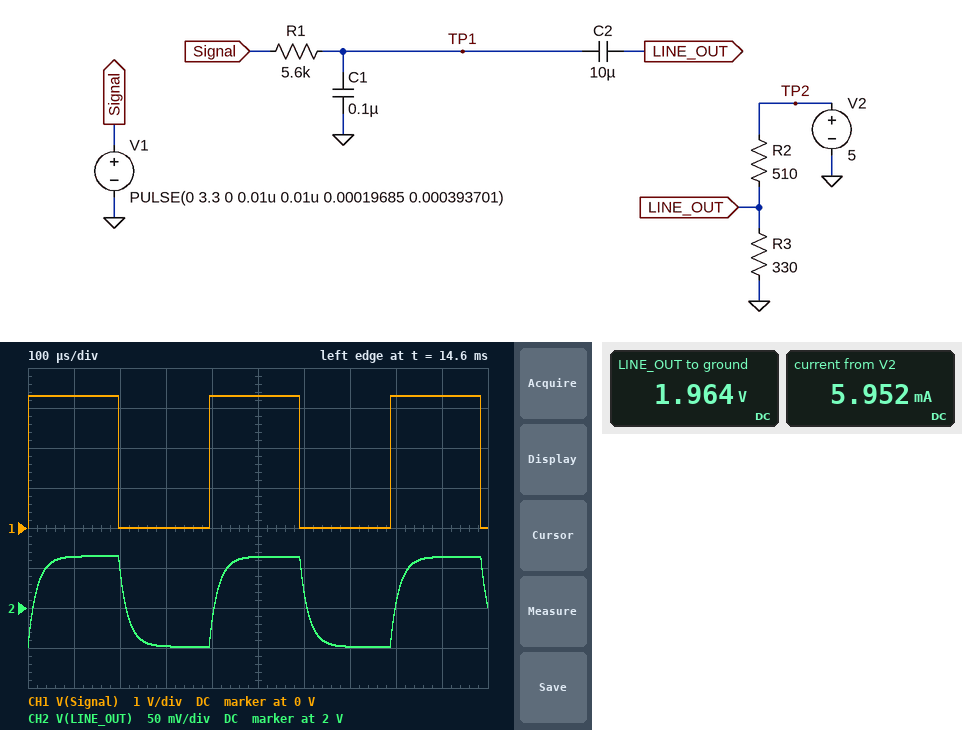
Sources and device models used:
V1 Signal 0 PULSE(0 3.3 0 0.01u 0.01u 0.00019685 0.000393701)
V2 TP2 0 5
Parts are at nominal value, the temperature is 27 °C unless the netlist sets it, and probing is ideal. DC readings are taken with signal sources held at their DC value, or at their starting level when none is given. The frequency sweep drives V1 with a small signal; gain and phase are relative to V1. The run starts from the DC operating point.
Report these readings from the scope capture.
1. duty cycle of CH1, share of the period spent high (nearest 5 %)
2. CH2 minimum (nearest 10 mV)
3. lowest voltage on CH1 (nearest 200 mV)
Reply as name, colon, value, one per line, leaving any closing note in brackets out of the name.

duty cycle of CH1, share of the period spent high: 50 %
CH2 minimum: 1.95 V
lowest voltage on CH1: 0 V
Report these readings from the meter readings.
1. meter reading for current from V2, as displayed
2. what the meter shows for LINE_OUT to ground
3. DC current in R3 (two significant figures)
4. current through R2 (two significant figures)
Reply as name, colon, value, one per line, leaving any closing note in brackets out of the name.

meter reading for current from V2, as displayed: 5.952 mA
what the meter shows for LINE_OUT to ground: 1.964 V
DC current in R3: 6.0 mA
current through R2: 6.0 mA
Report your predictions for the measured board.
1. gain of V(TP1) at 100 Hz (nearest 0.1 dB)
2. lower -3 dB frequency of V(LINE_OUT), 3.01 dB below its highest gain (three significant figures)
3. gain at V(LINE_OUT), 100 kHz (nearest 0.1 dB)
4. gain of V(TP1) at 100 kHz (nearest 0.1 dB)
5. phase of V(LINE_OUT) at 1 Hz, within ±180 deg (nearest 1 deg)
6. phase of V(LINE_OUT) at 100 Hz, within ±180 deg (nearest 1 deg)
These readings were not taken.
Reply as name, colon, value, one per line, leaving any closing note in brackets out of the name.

gain of V(TP1) at 100 Hz: -27.2 dB
lower -3 dB frequency of V(LINE_OUT), 3.01 dB below its highest gain: 2.72 Hz
gain at V(LINE_OUT), 100 kHz: -51.0 dB
gain of V(TP1) at 100 kHz: -51.0 dB
phase of V(LINE_OUT) at 1 Hz, within ±180 deg: 70 deg
phase of V(LINE_OUT) at 100 Hz, within ±180 deg: 1 deg
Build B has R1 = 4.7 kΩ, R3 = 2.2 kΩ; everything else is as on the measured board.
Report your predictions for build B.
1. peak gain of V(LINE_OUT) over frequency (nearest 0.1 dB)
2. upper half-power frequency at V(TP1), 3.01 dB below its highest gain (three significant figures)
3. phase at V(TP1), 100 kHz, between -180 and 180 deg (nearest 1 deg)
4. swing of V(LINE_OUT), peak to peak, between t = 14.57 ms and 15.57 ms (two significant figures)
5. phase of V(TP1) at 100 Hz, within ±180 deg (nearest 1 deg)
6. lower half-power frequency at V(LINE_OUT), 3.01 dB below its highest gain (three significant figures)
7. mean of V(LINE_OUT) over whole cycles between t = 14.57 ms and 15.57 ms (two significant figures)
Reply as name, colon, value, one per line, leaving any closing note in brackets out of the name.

peak gain of V(LINE_OUT) over frequency: -21.9 dB
upper half-power frequency at V(TP1), 3.01 dB below its highest gain: 3.11 Hz
phase at V(TP1), 100 kHz, between -180 and 180 deg: -88 deg
swing of V(LINE_OUT), peak to peak, between t = 14.57 ms and 15.57 ms: 260 mV
phase of V(TP1) at 100 Hz, within ±180 deg: -21 deg
lower half-power frequency at V(LINE_OUT), 3.01 dB below its highest gain: 3.08 Hz
mean of V(LINE_OUT) over whole cycles between t = 14.57 ms and 15.57 ms: 4.2 V
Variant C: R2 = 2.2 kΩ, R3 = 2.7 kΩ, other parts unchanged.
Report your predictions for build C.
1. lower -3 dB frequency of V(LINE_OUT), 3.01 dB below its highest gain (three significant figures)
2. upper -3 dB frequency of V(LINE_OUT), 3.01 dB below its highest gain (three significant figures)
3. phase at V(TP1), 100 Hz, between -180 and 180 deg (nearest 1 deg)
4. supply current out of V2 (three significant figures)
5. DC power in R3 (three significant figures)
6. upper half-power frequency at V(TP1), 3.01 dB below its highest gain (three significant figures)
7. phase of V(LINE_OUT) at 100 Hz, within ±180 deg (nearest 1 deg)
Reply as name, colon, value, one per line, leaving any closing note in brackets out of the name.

lower -3 dB frequency of V(LINE_OUT), 3.01 dB below its highest gain: 2.31 Hz
upper -3 dB frequency of V(LINE_OUT), 3.01 dB below its highest gain: 1.61 kHz
phase at V(TP1), 100 Hz, between -180 and 180 deg: -10 deg
supply current out of V2: 1.02 mA
DC power in R3: 2.81 mW
upper half-power frequency at V(TP1), 3.01 dB below its highest gain: 2.40 Hz
phase of V(LINE_OUT) at 100 Hz, within ±180 deg: -2 deg
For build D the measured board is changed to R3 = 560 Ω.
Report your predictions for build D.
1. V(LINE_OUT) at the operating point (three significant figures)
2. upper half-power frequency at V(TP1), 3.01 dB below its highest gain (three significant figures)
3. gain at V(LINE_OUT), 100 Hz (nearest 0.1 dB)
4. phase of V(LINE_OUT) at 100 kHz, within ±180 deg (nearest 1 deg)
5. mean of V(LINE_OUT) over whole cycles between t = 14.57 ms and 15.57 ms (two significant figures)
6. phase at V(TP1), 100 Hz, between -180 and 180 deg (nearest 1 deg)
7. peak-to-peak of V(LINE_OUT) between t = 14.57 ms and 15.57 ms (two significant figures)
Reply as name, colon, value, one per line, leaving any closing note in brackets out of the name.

V(LINE_OUT) at the operating point: 2.62 V
upper half-power frequency at V(TP1), 3.01 dB below its highest gain: 2.69 Hz
gain at V(LINE_OUT), 100 Hz: -26.9 dB
phase of V(LINE_OUT) at 100 kHz, within ±180 deg: -86 deg
mean of V(LINE_OUT) over whole cycles between t = 14.57 ms and 15.57 ms: 2.7 V
phase at V(TP1), 100 Hz, between -180 and 180 deg: -30 deg
peak-to-peak of V(LINE_OUT) between t = 14.57 ms and 15.57 ms: 150 mV
